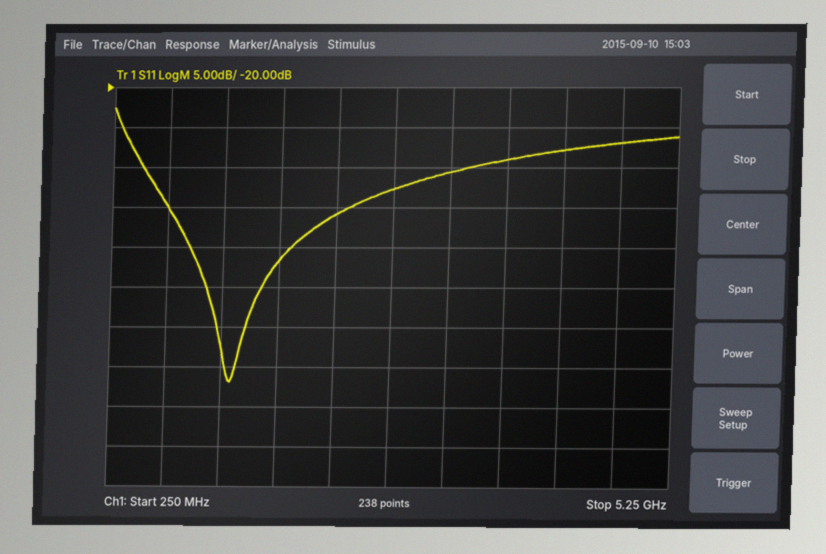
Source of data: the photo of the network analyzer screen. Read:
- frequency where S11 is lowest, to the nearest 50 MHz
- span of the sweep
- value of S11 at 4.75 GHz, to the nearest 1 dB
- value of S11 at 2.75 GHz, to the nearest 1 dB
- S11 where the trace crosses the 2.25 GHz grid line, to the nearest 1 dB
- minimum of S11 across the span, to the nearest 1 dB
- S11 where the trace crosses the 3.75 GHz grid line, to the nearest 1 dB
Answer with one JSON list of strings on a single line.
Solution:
["1.35 GHz", "5 GHz", "-27 dB", "-33 dB", "-36 dB", "-57 dB", "-29 dB"]
